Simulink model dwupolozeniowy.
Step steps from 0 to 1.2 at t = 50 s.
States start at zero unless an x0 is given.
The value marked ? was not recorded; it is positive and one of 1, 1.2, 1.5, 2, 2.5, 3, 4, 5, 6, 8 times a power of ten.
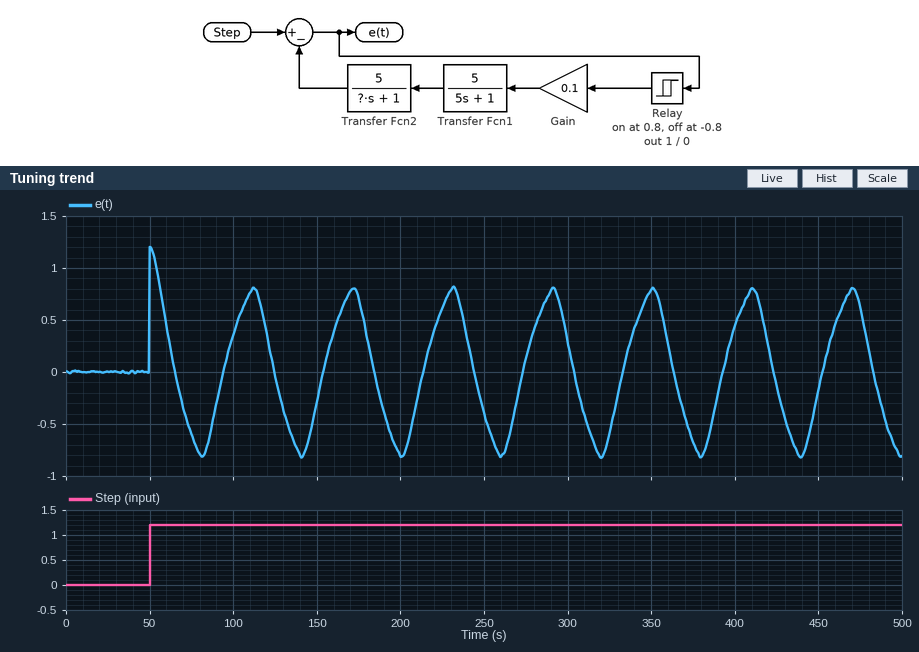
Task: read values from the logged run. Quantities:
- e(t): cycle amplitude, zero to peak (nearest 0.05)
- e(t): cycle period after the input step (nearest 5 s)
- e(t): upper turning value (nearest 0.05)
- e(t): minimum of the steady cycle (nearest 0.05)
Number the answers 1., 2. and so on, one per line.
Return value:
1. 0.80
2. 60 s
3. 0.80
4. -0.80
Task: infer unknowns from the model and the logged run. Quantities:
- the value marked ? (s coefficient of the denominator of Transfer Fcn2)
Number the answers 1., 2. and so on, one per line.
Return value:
1. 15
